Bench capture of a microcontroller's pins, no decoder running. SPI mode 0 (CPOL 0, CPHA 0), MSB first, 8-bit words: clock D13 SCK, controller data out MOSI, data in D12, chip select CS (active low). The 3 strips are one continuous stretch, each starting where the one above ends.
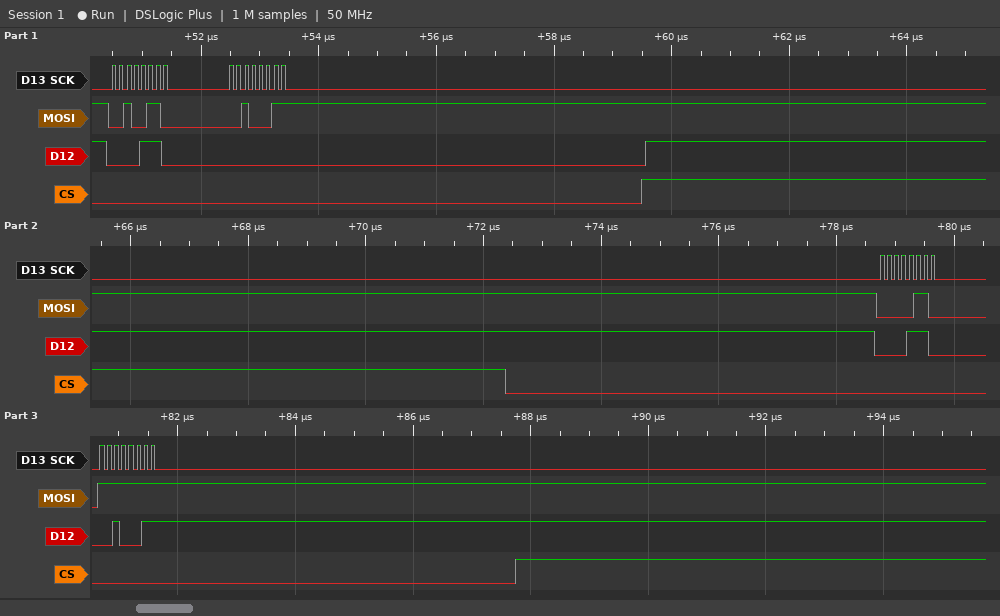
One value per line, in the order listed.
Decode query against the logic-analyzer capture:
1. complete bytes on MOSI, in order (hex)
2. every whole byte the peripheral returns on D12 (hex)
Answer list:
0x26 0x23 0x06 0xFF
0x0E 0x00 0x0E 0x23
